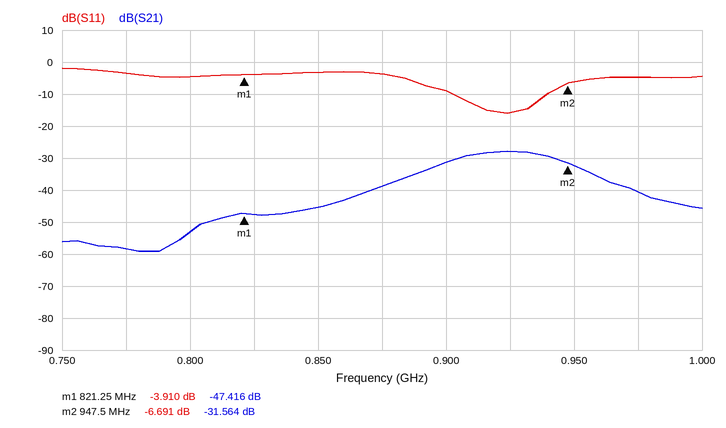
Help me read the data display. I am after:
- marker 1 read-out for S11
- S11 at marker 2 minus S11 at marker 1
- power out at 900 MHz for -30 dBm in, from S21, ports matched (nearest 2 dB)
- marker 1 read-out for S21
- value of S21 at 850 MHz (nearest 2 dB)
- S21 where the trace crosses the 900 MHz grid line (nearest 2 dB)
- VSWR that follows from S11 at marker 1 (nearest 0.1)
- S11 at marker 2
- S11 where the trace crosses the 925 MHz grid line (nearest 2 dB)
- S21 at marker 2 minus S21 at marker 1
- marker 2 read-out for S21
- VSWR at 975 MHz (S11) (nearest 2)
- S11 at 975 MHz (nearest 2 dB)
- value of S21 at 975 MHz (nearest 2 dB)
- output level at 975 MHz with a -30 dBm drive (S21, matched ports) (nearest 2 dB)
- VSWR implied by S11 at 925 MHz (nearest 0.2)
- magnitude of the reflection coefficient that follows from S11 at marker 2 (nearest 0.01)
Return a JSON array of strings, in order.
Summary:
["-3.910 dB", "-2.781 dB", "-62 dBm", "-47.416 dB", "-46 dB", "-32 dB", "4.5", "-6.691 dB", "-16 dB", "15.852 dB", "-31.564 dB", "4", "-4 dB", "-40 dB", "-70 dBm", "1.4", "0.46"]
